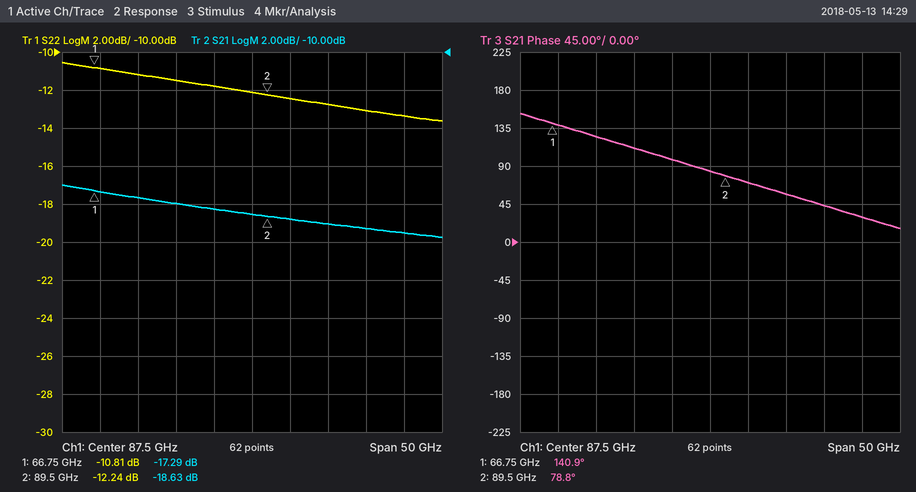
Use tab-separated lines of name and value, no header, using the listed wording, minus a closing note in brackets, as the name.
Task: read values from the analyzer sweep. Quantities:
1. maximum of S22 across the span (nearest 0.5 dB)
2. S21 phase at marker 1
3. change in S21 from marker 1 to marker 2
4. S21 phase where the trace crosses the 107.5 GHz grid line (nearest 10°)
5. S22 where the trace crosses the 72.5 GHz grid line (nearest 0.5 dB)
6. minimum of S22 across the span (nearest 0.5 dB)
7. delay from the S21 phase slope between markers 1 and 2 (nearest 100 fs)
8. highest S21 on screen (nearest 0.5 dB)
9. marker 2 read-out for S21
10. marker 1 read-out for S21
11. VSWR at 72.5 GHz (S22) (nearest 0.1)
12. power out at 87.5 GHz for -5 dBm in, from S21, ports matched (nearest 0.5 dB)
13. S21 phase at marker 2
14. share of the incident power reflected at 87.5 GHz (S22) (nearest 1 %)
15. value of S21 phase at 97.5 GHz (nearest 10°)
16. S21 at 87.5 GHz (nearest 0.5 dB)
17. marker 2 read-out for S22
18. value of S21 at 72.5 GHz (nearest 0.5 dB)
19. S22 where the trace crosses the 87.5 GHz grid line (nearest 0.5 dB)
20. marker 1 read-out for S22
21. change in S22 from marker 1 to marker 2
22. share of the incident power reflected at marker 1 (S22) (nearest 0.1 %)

maximum of S22 across the span	-10.5 dB
S21 phase at marker 1	140.9°
change in S21 from marker 1 to marker 2	-1.34 dB
S21 phase where the trace crosses the 107.5 GHz grid line	30°
S22 where the trace crosses the 72.5 GHz grid line	-11.0 dB
minimum of S22 across the span	-13.5 dB
delay from the S21 phase slope between markers 1 and 2	7.6 ps
highest S21 on screen	-17.0 dB
marker 2 read-out for S21	-18.63 dB
marker 1 read-out for S21	-17.29 dB
VSWR at 72.5 GHz (S22)	1.8
power out at 87.5 GHz for -5 dBm in, from S21, ports matched	-23.5 dBm
S21 phase at marker 2	78.8°
share of the incident power reflected at 87.5 GHz (S22)	6 %
value of S21 phase at 97.5 GHz	60°
S21 at 87.5 GHz	-18.5 dB
marker 2 read-out for S22	-12.24 dB
value of S21 at 72.5 GHz	-17.5 dB
S22 where the trace crosses the 87.5 GHz grid line	-12.0 dB
marker 1 read-out for S22	-10.81 dB
change in S22 from marker 1 to marker 2	-1.43 dB
share of the incident power reflected at marker 1 (S22)	8.3 %
